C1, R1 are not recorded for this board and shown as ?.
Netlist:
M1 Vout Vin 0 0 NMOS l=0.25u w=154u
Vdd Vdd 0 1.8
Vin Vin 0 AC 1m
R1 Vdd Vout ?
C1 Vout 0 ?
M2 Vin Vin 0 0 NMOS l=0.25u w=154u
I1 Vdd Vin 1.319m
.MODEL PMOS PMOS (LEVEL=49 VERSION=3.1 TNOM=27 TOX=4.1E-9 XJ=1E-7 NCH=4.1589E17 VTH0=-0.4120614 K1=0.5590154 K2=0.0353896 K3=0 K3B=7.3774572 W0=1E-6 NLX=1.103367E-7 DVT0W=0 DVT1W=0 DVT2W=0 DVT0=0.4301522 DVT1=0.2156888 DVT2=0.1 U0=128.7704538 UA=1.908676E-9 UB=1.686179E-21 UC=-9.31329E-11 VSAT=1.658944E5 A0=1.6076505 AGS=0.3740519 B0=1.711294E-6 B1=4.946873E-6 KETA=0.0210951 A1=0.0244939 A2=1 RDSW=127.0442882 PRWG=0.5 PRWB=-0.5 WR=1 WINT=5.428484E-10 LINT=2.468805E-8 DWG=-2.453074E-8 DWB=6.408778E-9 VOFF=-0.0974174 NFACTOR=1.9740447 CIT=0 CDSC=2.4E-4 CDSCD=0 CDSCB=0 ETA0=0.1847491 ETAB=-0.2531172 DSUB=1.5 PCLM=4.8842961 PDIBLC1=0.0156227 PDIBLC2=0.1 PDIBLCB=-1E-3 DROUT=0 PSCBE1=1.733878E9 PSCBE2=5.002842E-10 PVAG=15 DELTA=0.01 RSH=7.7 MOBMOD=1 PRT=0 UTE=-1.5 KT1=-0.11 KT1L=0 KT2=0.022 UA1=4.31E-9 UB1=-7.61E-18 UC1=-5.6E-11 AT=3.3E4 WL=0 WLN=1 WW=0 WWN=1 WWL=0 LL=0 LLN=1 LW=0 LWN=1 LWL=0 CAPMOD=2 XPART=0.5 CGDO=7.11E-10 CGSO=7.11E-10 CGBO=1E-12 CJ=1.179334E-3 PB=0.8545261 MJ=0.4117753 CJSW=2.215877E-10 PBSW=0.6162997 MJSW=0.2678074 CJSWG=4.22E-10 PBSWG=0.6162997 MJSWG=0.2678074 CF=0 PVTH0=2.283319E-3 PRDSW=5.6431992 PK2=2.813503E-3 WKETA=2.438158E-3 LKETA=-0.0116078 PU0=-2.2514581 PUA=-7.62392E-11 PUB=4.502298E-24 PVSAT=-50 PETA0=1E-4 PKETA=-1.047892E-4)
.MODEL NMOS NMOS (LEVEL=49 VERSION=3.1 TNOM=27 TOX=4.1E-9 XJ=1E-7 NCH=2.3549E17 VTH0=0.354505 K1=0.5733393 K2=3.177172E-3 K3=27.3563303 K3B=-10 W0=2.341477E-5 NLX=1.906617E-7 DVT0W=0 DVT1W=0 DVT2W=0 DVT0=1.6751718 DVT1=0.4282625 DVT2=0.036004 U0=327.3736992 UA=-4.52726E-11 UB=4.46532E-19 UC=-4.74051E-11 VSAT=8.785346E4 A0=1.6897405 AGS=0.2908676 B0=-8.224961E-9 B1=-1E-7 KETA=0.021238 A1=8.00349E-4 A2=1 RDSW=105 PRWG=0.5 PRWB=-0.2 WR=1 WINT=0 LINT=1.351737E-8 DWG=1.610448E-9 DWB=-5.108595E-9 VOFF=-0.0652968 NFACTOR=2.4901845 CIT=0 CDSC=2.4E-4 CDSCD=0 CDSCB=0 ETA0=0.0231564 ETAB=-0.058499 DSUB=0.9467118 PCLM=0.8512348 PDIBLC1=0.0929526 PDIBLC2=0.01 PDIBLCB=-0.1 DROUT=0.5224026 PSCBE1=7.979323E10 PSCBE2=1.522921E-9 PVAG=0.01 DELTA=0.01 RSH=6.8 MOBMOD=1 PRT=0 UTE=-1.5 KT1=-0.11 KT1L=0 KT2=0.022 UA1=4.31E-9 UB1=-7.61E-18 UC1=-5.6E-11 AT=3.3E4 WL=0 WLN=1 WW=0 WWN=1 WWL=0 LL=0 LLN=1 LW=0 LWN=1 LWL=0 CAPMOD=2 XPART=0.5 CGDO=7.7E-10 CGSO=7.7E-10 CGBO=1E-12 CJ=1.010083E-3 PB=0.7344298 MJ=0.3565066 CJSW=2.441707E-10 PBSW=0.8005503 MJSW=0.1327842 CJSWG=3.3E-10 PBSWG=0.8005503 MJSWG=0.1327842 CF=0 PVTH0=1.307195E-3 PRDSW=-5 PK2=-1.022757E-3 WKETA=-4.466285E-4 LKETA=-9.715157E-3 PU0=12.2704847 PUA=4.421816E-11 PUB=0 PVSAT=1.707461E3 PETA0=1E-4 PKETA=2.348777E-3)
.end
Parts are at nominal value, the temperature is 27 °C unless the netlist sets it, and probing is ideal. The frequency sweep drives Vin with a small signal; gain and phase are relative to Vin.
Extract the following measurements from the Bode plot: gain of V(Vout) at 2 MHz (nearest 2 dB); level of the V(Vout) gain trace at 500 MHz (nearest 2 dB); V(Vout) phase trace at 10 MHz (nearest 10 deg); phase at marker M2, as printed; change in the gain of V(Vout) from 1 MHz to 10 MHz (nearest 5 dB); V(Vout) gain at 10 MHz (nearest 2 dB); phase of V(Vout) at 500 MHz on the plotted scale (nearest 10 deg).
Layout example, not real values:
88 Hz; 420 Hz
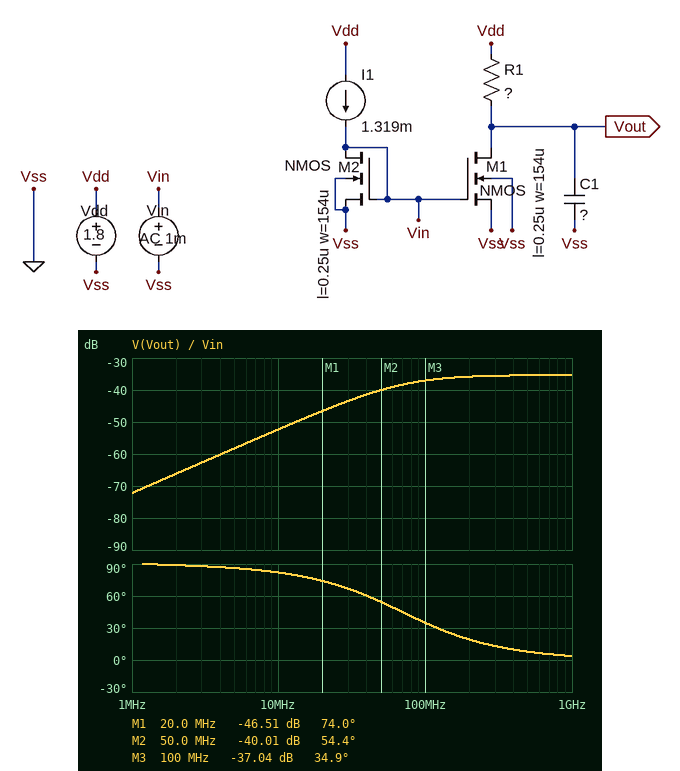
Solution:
-66 dB; -36 dB; 80 deg; 54.4 deg; 20 dB; -52 dB; 10 deg
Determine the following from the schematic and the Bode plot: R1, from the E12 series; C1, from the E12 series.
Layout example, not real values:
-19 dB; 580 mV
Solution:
330 Ω; 6.8 pF
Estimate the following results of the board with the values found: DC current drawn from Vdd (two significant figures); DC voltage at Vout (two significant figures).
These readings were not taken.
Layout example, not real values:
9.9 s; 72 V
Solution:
1.3 mA; 1.8 V
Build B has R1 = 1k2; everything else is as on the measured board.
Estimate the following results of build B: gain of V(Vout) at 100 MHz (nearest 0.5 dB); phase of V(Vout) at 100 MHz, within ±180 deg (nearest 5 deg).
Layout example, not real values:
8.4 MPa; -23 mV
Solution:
-35.5 dB; 10 deg
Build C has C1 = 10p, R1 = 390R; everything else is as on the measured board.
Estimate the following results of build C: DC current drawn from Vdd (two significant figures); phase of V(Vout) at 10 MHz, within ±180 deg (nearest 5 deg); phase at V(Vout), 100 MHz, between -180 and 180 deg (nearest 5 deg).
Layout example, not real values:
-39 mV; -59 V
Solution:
1.3 mA; 75 deg; 20 deg
